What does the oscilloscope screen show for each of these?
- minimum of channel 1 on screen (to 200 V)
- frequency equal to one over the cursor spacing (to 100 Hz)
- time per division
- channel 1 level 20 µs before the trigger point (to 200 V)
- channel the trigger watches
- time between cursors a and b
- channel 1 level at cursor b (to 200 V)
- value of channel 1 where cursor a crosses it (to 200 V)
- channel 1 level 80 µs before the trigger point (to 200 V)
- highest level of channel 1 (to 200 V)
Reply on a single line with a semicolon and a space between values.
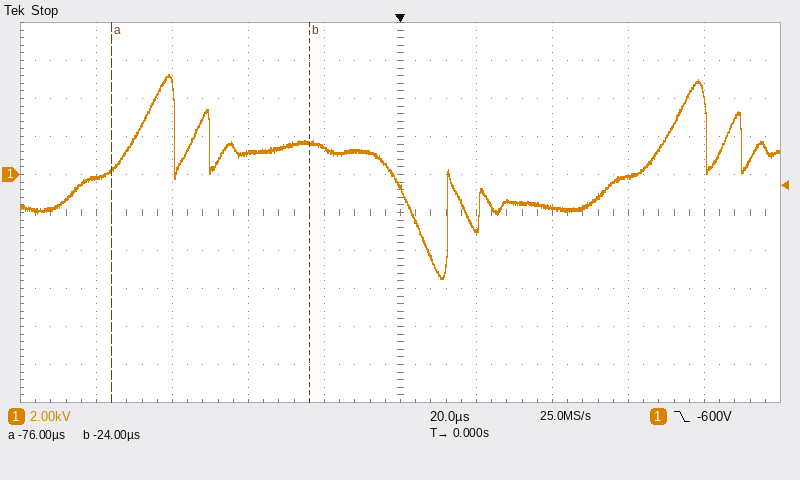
-5.4 kV; 19.2 kHz; 20 µs; 1.4 kV; channel 1; 52 µs; 1.6 kV; 200 V; -200 V; 5.2 kV
